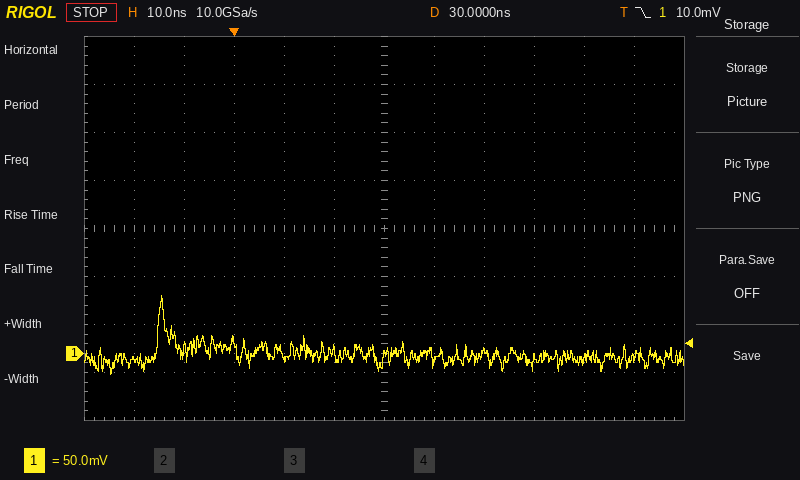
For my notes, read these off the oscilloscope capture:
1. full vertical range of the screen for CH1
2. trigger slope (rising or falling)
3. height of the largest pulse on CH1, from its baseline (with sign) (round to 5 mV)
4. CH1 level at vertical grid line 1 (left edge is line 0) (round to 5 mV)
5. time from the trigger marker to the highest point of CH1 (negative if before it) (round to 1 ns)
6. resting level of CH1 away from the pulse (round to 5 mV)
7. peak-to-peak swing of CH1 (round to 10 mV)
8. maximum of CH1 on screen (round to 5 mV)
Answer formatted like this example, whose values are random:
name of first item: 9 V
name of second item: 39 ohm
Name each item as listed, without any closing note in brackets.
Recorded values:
full vertical range of the screen for CH1: 400 mV
trigger slope: falling
height of the largest pulse on CH1, from its baseline (with sign): +65 mV
CH1 level at vertical grid line 1 (left edge is line 0): -5 mV
time from the trigger marker to the highest point of CH1 (negative if before it): -14 ns
resting level of CH1 away from the pulse: -5 mV
peak-to-peak swing of CH1: 80 mV
maximum of CH1 on screen: 60 mV
